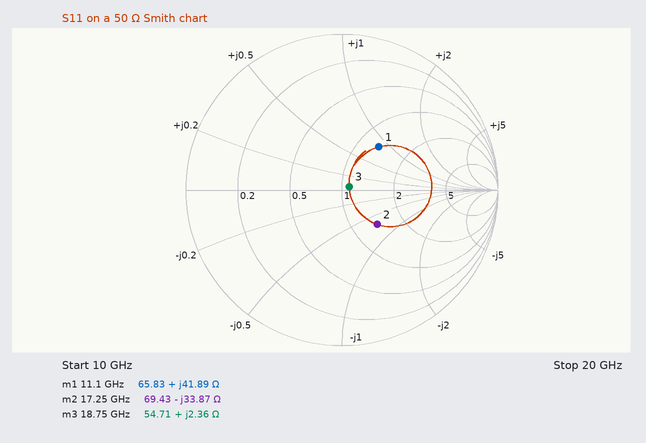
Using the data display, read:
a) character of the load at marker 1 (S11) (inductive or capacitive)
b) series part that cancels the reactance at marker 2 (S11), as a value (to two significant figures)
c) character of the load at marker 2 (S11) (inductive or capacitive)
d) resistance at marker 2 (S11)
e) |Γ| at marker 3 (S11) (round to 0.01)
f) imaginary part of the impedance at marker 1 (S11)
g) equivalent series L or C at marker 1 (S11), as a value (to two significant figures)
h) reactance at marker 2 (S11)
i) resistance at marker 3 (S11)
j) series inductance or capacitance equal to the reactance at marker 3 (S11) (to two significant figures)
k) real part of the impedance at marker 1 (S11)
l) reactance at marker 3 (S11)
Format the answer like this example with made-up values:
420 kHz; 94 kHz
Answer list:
inductive; 310 pH; capacitive; 69.43 Ω; 0.05; +41.89 Ω; 600 pH; -33.87 Ω; 54.71 Ω; 20 pH; 65.83 Ω; +2.36 Ω
